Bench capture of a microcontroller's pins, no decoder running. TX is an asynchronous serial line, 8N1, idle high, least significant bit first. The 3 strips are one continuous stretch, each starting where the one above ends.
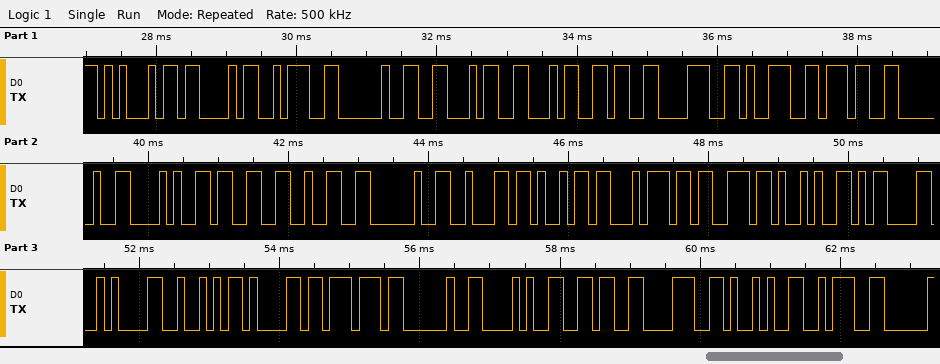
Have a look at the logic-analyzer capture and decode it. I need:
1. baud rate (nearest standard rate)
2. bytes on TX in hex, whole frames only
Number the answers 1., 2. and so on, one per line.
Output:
1. 9600 baud
2. 45 43 3A 20 46 46 36 38 39 37 20 28 33 32 20 62 69 74 73 29 0D 0A 52 61 77 20 28 36 38 29 3A
